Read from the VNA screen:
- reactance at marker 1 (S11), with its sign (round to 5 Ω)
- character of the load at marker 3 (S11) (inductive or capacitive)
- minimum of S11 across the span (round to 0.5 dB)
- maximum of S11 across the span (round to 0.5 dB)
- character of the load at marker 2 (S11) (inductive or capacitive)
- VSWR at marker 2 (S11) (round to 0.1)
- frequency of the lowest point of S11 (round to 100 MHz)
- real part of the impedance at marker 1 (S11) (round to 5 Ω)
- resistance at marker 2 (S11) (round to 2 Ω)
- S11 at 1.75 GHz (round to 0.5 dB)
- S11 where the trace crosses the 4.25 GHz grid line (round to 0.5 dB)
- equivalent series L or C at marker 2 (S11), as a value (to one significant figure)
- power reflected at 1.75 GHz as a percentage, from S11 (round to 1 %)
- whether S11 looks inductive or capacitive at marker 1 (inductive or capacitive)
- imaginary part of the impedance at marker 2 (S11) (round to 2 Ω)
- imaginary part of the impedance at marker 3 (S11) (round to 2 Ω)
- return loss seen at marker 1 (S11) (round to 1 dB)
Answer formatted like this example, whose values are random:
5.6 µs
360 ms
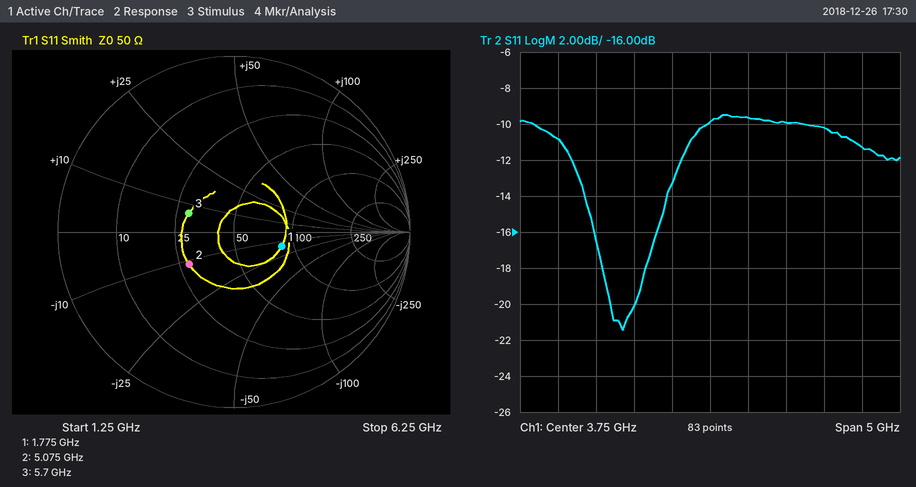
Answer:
-15 Ω
inductive
-21.5 dB
-9.5 dB
capacitive
1.9
2.6 GHz
85 Ω
28 Ω
-11.0 dB
-9.5 dB
3 pF
8 %
capacitive
-12 Ω
+6 Ω
11 dB
